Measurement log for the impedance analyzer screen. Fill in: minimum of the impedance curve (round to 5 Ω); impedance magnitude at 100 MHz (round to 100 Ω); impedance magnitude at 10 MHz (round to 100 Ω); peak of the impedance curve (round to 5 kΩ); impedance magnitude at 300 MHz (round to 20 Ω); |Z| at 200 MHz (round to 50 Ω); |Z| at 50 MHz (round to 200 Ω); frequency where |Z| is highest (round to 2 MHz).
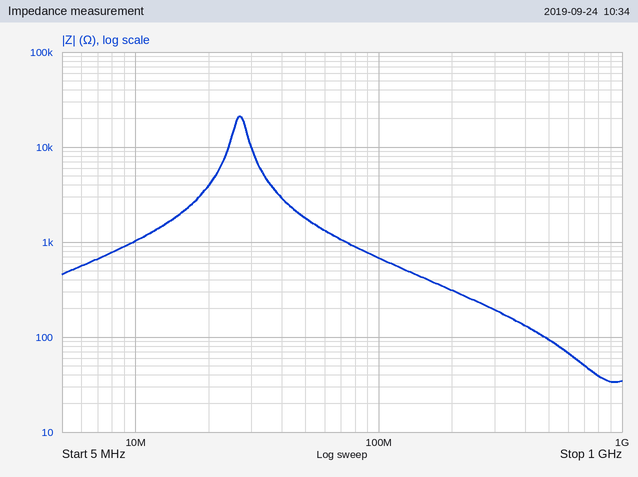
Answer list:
35 Ω
700 Ω
1.0 kΩ
20 kΩ
200 Ω
300 Ω
1.8 kΩ
26 MHz
